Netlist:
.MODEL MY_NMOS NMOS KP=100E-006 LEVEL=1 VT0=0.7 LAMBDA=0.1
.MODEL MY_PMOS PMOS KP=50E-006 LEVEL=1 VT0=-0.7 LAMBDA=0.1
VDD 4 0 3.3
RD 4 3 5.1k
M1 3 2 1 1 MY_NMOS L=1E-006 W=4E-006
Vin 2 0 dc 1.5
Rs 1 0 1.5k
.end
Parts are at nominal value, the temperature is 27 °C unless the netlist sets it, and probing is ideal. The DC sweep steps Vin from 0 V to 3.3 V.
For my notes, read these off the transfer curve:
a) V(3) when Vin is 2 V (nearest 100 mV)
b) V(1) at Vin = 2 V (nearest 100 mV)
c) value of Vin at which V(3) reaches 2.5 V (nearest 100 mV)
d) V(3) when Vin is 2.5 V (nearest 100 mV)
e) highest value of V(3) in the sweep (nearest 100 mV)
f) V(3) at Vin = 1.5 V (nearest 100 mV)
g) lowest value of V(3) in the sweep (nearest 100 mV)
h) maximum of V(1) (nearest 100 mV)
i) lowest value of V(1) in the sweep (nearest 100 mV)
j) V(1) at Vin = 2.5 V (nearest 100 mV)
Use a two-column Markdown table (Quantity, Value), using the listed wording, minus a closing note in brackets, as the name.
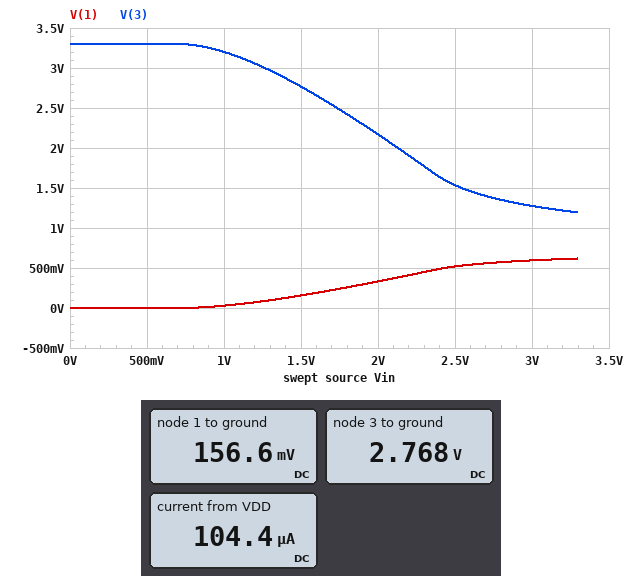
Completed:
| Quantity | Value |
|---|---|
| V(3) when Vin is 2 V | 2.2 V |
| V(1) at Vin = 2 V | 300 mV |
| value of Vin at which V(3) reaches 2.5 V | 1.7 V |
| V(3) when Vin is 2.5 V | 1.5 V |
| highest value of V(3) in the sweep | 3.3 V |
| V(3) at Vin = 1.5 V | 2.8 V |
| lowest value of V(3) in the sweep | 1.2 V |
| maximum of V(1) | 600 mV |
| lowest value of V(1) in the sweep | 0 V |
| V(1) at Vin = 2.5 V | 500 mV |
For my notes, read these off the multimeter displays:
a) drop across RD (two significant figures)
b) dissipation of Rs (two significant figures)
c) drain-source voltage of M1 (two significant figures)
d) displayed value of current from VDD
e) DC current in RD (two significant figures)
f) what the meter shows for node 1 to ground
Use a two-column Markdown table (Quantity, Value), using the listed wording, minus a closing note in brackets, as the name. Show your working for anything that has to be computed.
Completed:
| Quantity | Value |
|---|---|
| drop across RD | 3.3 V - 2.768 V = 530 mV |
| dissipation of Rs | (156.6 mV)^2 / 1.5 kΩ = 16 µW |
| drain-source voltage of M1 | 2.768 V - 156.6 mV = 2.6 V |
| displayed value of current from VDD | 104.4 µA |
| DC current in RD | (3.3 V - 2.768 V) / 5.1 kΩ = 100 µA |
| what the meter shows for node 1 to ground | 156.6 mV |
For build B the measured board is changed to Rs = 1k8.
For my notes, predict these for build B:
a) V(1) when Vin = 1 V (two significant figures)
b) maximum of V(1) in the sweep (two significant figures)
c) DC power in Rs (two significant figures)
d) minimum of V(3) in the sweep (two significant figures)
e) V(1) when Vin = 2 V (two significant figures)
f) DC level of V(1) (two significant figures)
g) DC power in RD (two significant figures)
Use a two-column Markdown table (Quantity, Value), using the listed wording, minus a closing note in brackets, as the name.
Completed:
| Quantity | Value |
|---|---|
| V(1) when Vin = 1 V | 34 mV |
| maximum of V(1) in the sweep | 710 mV |
| DC power in Rs | 17 µW |
| minimum of V(3) in the sweep | 1.3 V |
| V(1) when Vin = 2 V | 370 mV |
| DC level of V(1) | 180 mV |
| DC power in RD | 49 µW |
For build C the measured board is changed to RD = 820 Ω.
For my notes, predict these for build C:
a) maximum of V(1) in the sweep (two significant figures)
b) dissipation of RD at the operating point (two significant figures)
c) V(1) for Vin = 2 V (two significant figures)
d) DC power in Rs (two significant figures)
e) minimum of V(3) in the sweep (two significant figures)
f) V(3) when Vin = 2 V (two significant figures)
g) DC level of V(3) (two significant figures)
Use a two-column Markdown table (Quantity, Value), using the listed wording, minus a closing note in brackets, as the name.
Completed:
| Quantity | Value |
|---|---|
| maximum of V(1) in the sweep | 960 mV |
| dissipation of RD at the operating point | 9.4 µW |
| V(1) for Vin = 2 V | 350 mV |
| DC power in Rs | 17 µW |
| minimum of V(3) in the sweep | 2.8 V |
| V(3) when Vin = 2 V | 3.1 V |
| DC level of V(3) | 3.2 V |
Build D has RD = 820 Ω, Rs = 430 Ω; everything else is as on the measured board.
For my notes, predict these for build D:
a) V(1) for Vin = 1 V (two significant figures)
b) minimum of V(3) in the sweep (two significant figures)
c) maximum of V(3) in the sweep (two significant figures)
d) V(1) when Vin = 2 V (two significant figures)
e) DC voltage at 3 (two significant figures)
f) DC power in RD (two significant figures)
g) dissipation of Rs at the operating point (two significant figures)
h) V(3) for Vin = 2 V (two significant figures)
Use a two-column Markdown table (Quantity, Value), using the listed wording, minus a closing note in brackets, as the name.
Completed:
| Quantity | Value |
|---|---|
| V(1) for Vin = 1 V | 9.6 mV |
| minimum of V(3) in the sweep | 2.4 V |
| maximum of V(3) in the sweep | 3.3 V |
| V(1) when Vin = 2 V | 150 mV |
| DC voltage at 3 | 3.2 V |
| DC power in RD | 17 µW |
| dissipation of Rs at the operating point | 8.8 µW |
| V(3) for Vin = 2 V | 3.0 V |
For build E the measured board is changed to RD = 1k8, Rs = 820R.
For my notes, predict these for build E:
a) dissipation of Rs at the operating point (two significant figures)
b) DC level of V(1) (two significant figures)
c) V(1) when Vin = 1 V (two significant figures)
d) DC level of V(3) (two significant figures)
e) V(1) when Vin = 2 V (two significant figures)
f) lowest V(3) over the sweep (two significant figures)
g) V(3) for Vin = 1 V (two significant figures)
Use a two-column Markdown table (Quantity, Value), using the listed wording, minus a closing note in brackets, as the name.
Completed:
| Quantity | Value |
|---|---|
| dissipation of Rs at the operating point | 13 µW |
| DC level of V(1) | 100 mV |
| V(1) when Vin = 1 V | 17 mV |
| DC level of V(3) | 3.1 V |
| V(1) when Vin = 2 V | 230 mV |
| lowest V(3) over the sweep | 1.9 V |
| V(3) for Vin = 1 V | 3.3 V |
